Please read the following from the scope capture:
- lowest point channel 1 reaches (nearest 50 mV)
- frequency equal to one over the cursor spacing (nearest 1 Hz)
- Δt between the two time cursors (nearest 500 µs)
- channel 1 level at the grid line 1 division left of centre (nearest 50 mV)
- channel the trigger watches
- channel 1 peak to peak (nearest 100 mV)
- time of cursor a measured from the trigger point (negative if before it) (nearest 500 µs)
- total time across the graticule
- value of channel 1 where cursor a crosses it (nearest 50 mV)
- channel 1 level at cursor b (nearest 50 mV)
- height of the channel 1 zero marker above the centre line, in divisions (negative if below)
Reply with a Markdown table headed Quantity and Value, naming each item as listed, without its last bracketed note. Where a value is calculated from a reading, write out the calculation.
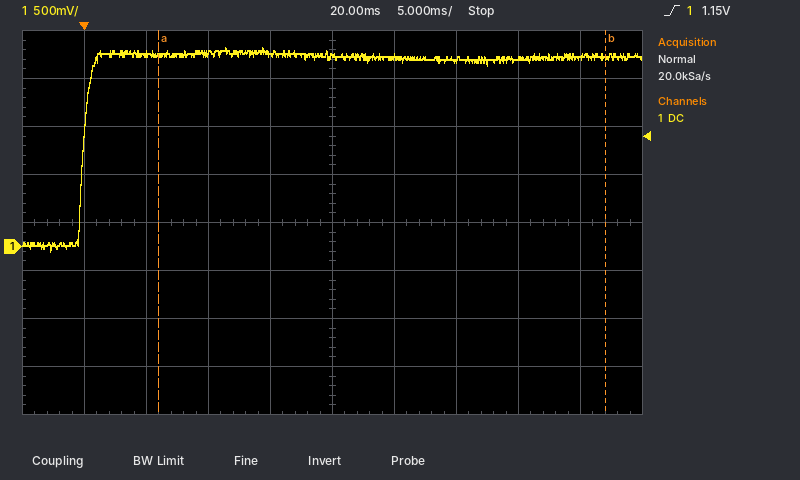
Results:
| Quantity | Value |
|---|---|
| lowest point channel 1 reaches | -50 mV |
| frequency equal to one over the cursor spacing | 1 / 36.0 ms ≈ 28 Hz |
| Δt between the two time cursors | 36.0 ms |
| channel 1 level at the grid line 1 division left of centre | 2.00 V |
| channel the trigger watches | channel 1 |
| channel 1 peak to peak | 2.10 V |
| time of cursor a measured from the trigger point (negative if before it) | +6.0 ms |
| total time across the graticule | 50 ms |
| value of channel 1 where cursor a crosses it | 2.00 V |
| channel 1 level at cursor b | 2.00 V |
| height of the channel 1 zero marker above the centre line, in divisions | -0.5 div |
